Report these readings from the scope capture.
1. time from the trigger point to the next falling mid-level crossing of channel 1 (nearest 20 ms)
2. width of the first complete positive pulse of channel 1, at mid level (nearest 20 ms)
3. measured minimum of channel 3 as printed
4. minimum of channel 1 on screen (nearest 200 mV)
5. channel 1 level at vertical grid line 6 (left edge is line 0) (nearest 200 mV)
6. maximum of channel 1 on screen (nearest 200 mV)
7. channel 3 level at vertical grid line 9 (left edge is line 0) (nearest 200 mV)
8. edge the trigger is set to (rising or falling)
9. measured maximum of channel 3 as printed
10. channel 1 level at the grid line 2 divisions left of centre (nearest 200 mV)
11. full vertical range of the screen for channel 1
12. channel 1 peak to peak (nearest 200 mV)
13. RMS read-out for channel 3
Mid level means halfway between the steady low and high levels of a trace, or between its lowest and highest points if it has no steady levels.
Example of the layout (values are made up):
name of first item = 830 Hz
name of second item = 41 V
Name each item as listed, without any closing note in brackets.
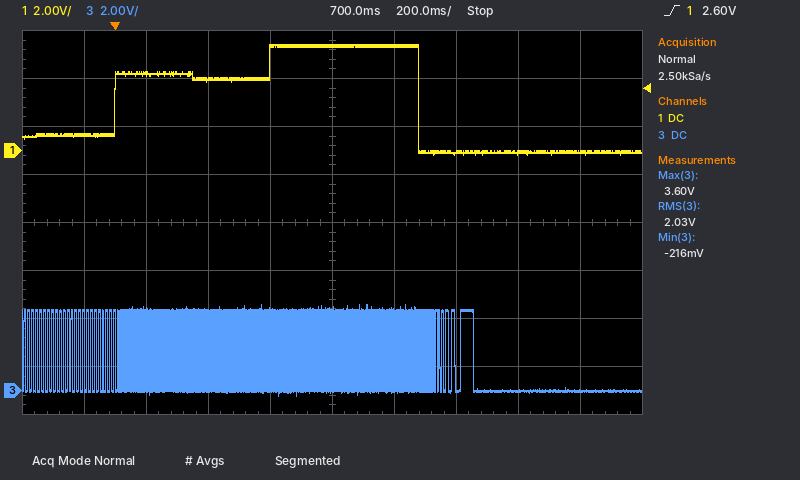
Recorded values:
time from the trigger point to the next falling mid-level crossing of channel 1 = 980 ms
width of the first complete positive pulse of channel 1, at mid level = 980 ms
measured minimum of channel 3 as printed = -216 mV
minimum of channel 1 on screen = -200 mV
channel 1 level at vertical grid line 6 (left edge is line 0) = 4.4 V
maximum of channel 1 on screen = 4.4 V
channel 3 level at vertical grid line 9 (left edge is line 0) = 0.0 V
edge the trigger is set to = rising
measured maximum of channel 3 as printed = 3.60 V
channel 1 level at the grid line 2 divisions left of centre = 3.0 V
full vertical range of the screen for channel 1 = 16 V
channel 1 peak to peak = 4.6 V
RMS read-out for channel 3 = 2.03 V
